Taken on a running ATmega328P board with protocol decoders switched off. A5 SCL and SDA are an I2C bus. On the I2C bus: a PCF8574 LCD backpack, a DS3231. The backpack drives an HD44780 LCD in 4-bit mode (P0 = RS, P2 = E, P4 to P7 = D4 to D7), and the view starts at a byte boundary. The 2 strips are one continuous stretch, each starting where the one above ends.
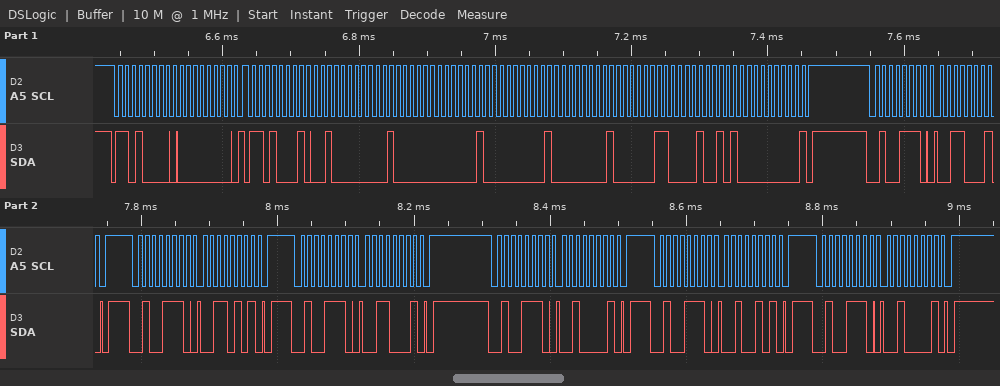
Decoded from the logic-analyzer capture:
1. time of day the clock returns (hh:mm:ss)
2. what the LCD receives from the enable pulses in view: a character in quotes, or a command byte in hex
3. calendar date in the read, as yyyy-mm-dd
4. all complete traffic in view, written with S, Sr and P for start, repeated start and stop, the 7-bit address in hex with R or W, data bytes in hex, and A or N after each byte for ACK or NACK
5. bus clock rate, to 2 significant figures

02:20:20
'2'
2025-06-01
S 68W A 00 A Sr 68R A 20 A 20 A 02 A 01 A 01 A 06 A 25 A 00 N P S 27W A 31 A P S 27W A 35 A P S 27W A 31 A P S 27W A 21 A P S 27W A 25 A P S 27W A 21 A P
100 kHz
